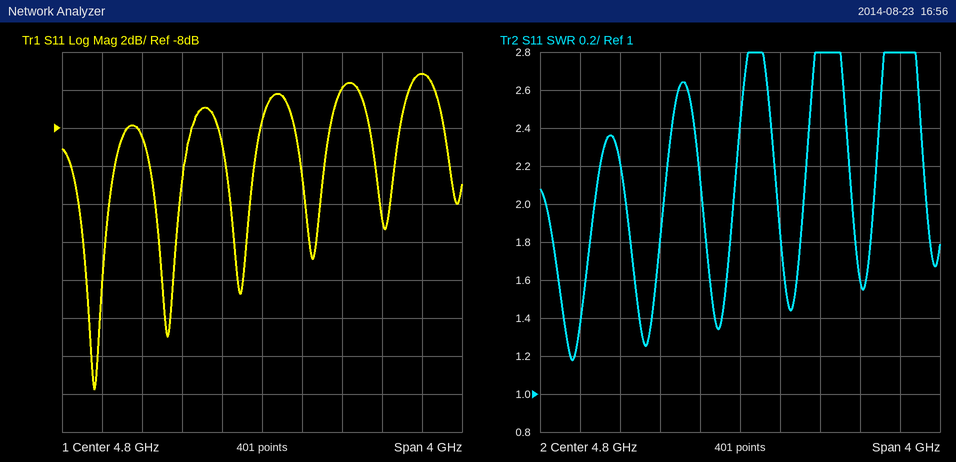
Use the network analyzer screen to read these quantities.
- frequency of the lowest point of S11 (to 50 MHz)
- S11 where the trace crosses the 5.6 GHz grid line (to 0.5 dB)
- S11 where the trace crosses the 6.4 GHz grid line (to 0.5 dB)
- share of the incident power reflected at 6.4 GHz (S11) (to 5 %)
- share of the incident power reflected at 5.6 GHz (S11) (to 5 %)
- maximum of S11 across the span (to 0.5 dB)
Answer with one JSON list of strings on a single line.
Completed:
["3.10 GHz", "-6.0 dB", "-5.0 dB", "30 %", "25 %", "-5.0 dB"]
